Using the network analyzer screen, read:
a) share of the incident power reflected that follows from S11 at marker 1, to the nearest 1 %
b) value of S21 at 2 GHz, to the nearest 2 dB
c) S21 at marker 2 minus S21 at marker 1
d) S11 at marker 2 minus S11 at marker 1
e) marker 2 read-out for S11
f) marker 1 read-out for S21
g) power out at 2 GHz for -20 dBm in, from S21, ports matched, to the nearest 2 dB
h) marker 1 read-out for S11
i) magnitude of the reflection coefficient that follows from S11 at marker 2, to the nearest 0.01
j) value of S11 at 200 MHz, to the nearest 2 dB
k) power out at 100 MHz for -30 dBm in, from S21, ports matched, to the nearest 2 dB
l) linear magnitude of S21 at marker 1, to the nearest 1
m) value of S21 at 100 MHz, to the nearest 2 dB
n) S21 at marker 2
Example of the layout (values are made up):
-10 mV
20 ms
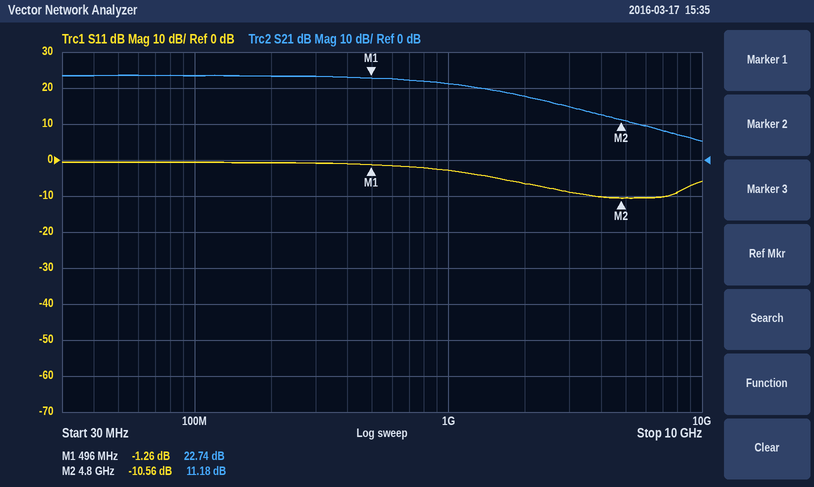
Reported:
75 %
18 dB
-11.56 dB
-9.30 dB
-10.56 dB
22.74 dB
-2 dBm
-1.26 dB
0.30
0 dB
-6 dBm
14
24 dB
11.18 dB
